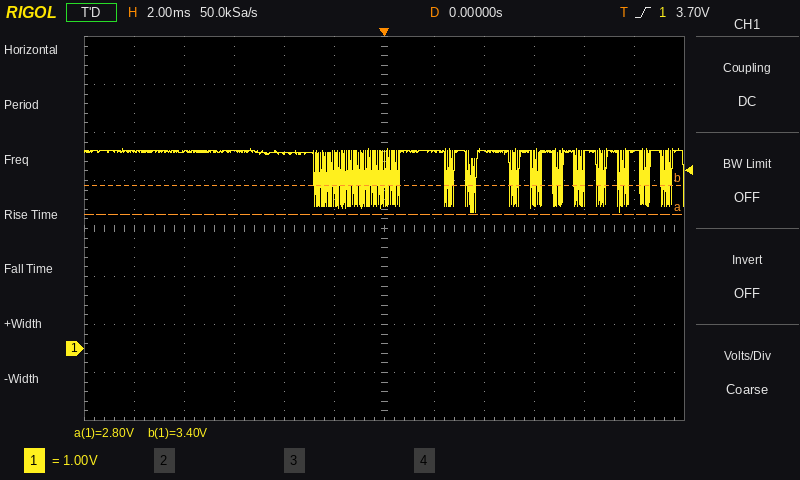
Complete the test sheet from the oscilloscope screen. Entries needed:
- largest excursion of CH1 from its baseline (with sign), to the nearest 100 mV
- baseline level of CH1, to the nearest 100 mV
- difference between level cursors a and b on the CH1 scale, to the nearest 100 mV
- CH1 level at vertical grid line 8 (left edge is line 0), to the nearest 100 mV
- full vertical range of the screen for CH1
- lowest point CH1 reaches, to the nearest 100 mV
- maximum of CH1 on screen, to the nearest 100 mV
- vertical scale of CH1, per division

-1.3 V
4.1 V
600 mV
4.1 V
8 V
2.8 V
4.2 V
1 V
